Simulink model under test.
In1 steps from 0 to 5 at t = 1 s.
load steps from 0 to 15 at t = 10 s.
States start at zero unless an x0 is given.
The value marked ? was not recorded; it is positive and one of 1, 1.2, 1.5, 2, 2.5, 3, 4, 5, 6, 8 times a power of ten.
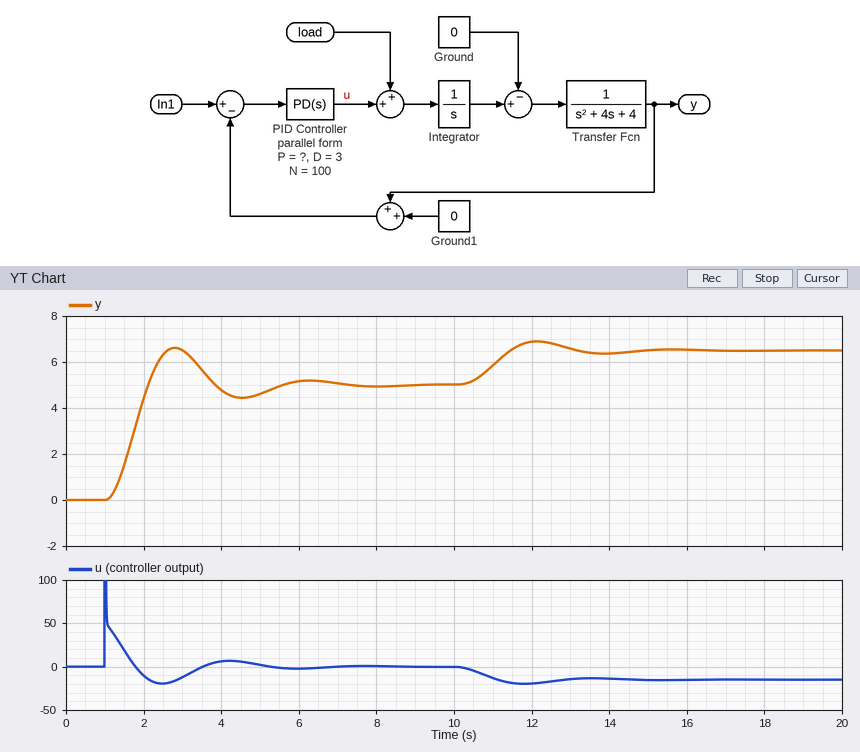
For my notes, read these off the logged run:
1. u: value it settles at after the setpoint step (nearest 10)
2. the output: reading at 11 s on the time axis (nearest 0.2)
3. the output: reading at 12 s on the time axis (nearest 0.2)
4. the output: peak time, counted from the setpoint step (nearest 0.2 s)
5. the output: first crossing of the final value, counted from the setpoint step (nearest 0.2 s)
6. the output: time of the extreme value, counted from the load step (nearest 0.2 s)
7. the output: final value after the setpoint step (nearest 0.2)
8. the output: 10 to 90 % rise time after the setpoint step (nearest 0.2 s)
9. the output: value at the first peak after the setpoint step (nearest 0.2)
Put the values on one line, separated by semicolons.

0; 5.8; 6.8; 1.8 s; 1.2 s; 2.2 s; 5.0; 0.8 s; 6.6
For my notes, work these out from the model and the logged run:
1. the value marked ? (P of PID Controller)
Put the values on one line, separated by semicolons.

10
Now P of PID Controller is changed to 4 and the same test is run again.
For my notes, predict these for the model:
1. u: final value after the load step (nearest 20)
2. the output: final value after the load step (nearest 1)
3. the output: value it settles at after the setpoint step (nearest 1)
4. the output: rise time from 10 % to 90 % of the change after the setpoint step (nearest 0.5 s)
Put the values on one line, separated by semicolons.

-20; 9; 5; 1.5 s
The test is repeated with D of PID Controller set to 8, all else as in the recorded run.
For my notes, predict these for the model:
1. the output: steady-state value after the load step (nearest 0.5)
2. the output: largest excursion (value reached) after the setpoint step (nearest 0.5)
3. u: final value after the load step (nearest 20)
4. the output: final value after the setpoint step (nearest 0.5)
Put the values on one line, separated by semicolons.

6.5; 5.5; -20; 5.0
